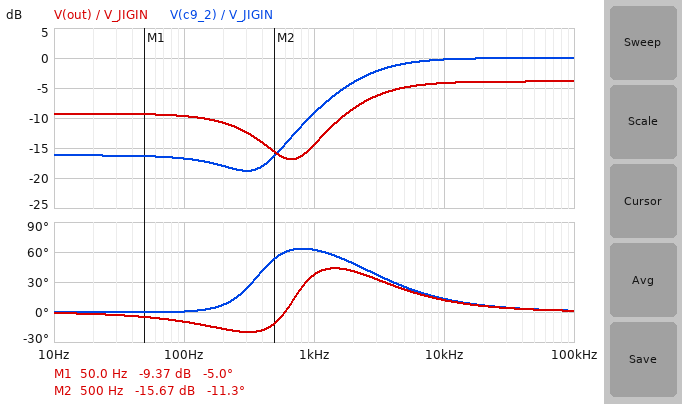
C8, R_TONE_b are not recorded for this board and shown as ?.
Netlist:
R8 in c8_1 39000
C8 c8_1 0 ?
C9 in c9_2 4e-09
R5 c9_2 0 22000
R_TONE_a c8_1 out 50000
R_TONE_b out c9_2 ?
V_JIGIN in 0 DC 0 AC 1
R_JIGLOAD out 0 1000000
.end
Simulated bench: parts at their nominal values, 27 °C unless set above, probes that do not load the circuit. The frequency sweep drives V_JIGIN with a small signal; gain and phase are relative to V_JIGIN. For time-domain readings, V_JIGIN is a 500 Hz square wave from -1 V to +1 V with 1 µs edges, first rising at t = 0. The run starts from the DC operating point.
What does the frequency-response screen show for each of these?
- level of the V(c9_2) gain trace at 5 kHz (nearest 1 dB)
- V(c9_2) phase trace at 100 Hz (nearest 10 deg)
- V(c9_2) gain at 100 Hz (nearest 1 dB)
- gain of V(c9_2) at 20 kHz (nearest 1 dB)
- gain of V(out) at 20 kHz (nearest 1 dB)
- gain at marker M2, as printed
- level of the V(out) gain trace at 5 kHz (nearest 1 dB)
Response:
-1 dB
0 deg
-17 dB
0 dB
-4 dB
-15.67 dB
-5 dB
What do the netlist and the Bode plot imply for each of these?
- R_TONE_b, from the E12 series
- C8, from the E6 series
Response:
27 kΩ
15 nF
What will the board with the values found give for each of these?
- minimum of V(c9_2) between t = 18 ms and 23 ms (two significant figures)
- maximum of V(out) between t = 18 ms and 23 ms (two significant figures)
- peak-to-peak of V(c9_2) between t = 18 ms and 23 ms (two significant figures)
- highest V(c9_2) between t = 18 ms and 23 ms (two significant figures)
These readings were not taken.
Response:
-1.9 V
980 mV
3.7 V
1.9 V
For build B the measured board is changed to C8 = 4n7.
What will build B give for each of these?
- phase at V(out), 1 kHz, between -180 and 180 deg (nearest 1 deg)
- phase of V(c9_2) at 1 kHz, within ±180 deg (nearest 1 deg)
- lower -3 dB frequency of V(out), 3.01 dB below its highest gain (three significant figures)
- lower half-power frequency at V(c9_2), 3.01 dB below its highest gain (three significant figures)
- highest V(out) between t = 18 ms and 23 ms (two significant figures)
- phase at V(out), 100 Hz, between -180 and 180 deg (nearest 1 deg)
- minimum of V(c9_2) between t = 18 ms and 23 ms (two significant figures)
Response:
12 deg
50 deg
2.50 kHz
2.66 kHz
930 mV
0 deg
-1.8 V
